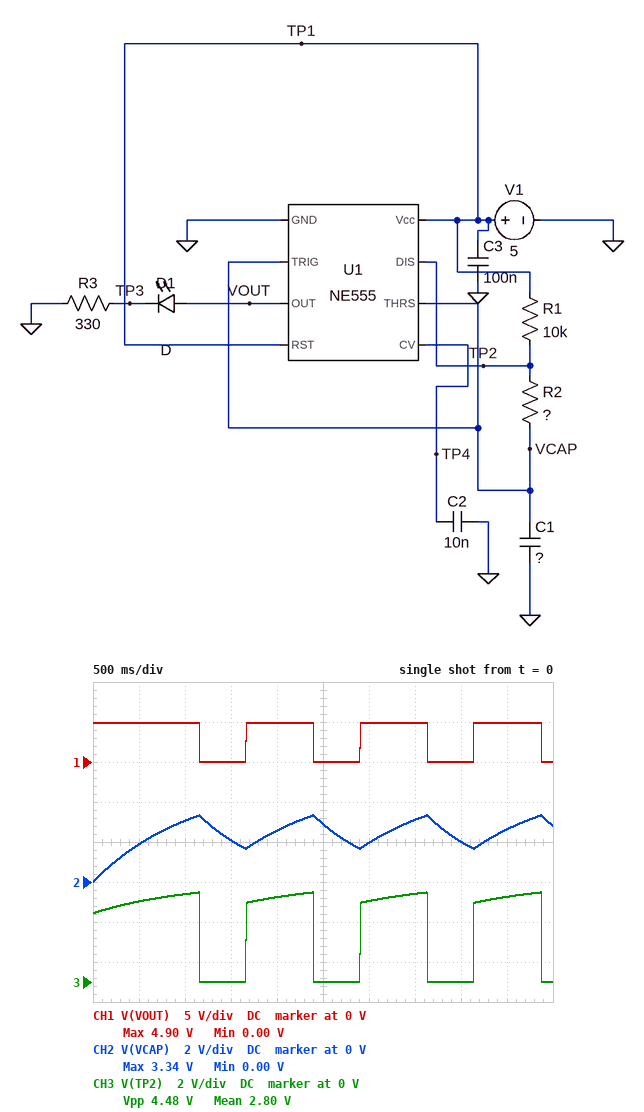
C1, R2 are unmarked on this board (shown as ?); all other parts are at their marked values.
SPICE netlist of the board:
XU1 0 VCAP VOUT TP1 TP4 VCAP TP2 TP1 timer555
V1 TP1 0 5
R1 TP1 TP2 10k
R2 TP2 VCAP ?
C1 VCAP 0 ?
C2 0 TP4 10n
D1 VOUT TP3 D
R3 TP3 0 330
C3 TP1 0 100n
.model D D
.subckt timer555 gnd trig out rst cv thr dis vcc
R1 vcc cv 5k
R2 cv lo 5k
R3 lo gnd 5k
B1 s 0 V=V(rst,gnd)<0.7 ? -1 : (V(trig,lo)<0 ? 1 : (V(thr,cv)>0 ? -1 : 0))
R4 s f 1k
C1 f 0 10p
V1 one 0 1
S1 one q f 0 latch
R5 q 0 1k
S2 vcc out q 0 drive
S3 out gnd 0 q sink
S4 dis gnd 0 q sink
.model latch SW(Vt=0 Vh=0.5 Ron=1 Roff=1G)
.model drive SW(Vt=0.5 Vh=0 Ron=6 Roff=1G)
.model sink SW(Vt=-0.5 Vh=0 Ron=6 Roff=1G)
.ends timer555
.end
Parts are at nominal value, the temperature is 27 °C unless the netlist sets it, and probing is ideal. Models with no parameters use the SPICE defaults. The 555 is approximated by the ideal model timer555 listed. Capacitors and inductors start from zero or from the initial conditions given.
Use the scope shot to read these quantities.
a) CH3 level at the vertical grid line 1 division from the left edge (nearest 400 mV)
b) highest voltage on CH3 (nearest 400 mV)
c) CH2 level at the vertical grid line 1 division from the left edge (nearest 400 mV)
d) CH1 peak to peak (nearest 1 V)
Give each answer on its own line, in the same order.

4.0 V
4.4 V
2.0 V
5 V
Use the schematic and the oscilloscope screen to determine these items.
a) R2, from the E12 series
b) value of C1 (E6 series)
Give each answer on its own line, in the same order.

22 kΩ
33 µF
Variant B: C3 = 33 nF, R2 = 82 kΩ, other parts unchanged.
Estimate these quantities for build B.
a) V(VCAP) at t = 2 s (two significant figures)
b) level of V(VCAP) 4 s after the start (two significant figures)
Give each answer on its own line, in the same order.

2.4 V
2.6 V
